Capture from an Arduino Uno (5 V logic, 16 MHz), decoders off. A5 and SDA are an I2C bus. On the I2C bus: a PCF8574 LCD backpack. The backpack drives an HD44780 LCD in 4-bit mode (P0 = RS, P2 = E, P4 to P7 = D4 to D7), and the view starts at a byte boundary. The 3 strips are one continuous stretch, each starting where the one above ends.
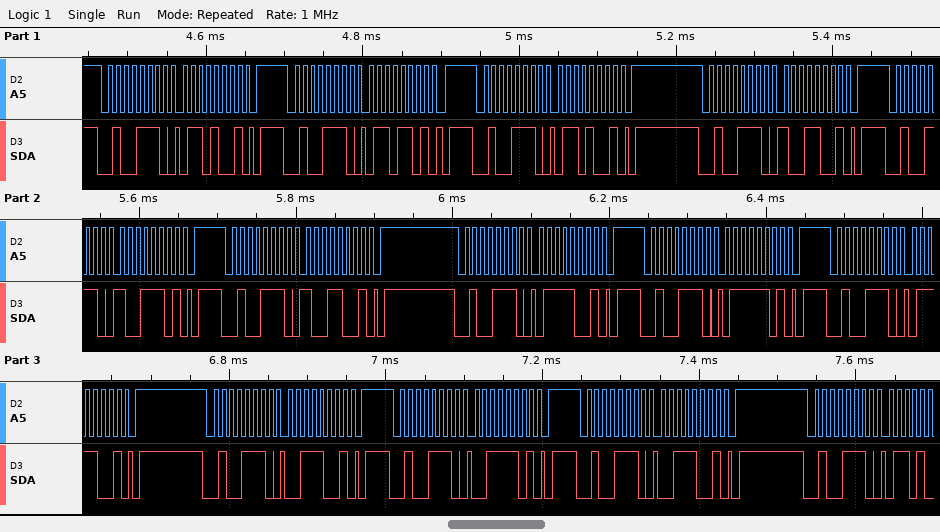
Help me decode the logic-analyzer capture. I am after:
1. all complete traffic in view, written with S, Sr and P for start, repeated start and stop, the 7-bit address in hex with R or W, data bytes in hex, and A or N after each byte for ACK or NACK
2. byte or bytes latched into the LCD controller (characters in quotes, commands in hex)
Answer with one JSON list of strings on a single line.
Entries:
["S 27W A 69 A P S 27W A 6D A P S 27W A 69 A P S 27W A 99 A P S 27W A 9D A P S 27W A 99 A P S 27W A 79 A P S 27W A 7D A P S 27W A 79 A P S 27W A 39 A P S 27W A 3D A P S 27W A 39 A P S 27W A", "'i' 's'"]
